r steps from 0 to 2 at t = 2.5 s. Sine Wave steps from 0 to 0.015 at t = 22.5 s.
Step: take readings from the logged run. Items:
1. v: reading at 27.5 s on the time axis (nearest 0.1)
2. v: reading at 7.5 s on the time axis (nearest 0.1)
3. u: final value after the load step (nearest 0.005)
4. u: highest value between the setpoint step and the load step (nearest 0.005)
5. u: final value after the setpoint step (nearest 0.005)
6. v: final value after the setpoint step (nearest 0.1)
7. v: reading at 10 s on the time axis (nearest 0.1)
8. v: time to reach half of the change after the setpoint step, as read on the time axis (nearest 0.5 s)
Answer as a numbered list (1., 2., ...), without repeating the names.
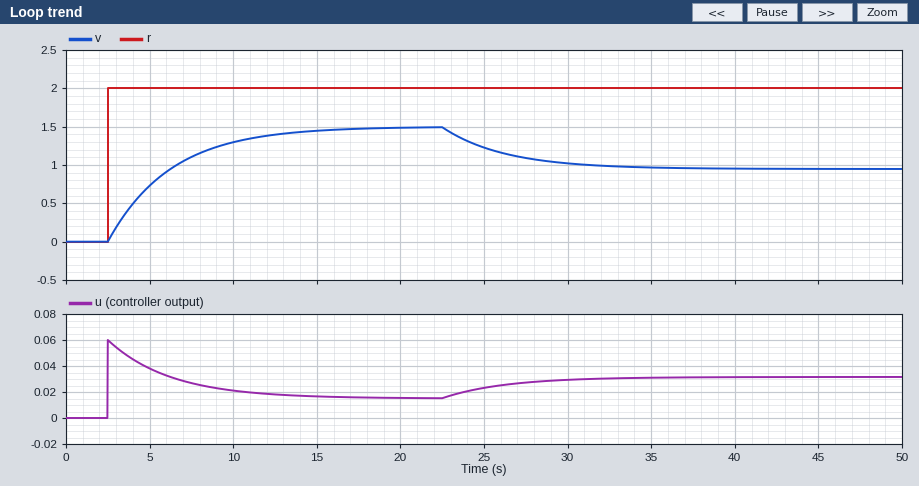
1. 1.1
2. 1.1
3. 0.030
4. 0.060
5. 0.015
6. 1.5
7. 1.3
8. 5.0 s
